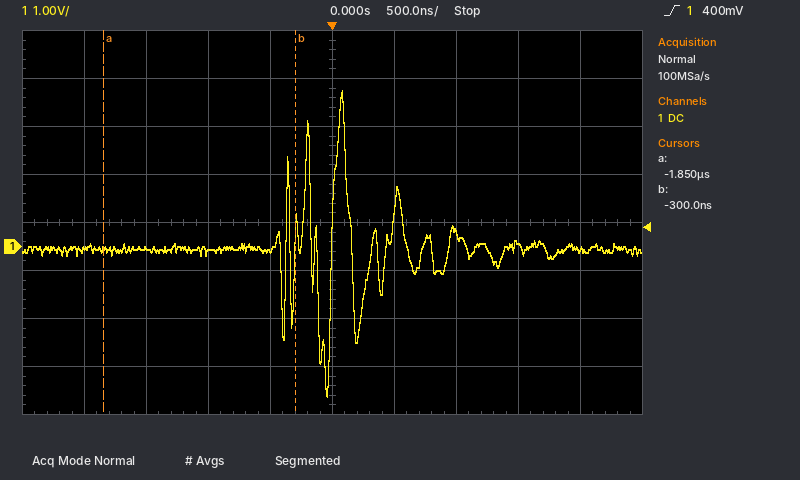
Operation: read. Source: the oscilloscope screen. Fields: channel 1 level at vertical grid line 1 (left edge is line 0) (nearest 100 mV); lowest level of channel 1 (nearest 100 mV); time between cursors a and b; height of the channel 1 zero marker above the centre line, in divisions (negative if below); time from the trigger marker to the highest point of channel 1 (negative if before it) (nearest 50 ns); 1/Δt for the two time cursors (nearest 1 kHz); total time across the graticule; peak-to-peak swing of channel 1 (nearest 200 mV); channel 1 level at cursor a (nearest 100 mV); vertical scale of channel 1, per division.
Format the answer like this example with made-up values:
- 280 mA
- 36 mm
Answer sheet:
- -100 mV
- -3.1 V
- 1.55 µs
- -0.5 div
- +100 ns
- 645 kHz
- 5 µs
- 6.4 V
- -100 mV
- 1 V
